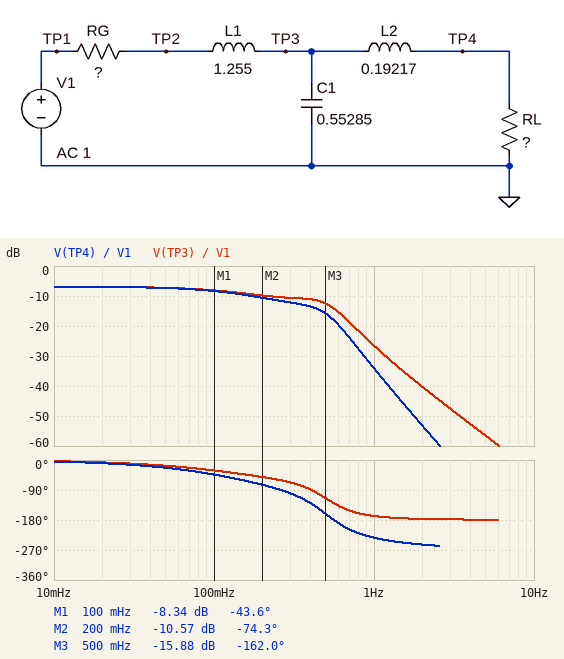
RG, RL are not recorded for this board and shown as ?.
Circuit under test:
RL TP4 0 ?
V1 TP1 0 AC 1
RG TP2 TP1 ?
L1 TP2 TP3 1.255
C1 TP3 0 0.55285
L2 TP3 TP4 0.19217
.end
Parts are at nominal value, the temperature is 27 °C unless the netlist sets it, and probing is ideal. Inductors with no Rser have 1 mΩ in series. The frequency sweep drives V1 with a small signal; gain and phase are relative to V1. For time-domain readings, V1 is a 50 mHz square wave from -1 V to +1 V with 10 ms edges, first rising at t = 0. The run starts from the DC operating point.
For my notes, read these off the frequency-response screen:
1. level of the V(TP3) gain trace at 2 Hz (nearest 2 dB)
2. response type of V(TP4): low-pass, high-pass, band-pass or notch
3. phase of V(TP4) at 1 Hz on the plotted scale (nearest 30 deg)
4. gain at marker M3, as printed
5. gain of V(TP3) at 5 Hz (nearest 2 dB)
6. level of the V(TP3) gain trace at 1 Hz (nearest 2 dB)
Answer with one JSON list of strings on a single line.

["-40 dB", "low-pass", "-240 deg", "-15.88 dB", "-56 dB", "-26 dB"]
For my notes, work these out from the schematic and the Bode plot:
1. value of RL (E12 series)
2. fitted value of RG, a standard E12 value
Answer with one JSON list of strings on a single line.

["0.56 Ω", "0.68 Ω"]
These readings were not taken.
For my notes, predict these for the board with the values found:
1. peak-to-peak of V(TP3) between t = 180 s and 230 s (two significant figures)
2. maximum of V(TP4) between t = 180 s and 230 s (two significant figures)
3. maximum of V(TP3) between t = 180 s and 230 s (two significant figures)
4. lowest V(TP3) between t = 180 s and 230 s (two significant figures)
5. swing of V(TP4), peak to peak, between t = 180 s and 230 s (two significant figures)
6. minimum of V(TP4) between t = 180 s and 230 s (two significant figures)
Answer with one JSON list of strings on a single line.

["900 mV", "450 mV", "450 mV", "-450 mV", "900 mV", "-450 mV"]
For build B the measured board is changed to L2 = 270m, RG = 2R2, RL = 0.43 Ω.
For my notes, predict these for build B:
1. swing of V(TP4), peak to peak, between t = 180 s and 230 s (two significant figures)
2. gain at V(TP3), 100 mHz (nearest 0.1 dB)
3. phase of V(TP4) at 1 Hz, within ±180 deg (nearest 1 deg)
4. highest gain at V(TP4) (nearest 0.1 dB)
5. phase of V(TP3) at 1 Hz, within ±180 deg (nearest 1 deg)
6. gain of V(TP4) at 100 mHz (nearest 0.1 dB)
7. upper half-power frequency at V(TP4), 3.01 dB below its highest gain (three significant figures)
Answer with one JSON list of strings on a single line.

["400 mV", "-15.3 dB", "123 deg", "-15.4 dB", "-161 deg", "-15.9 dB", "498 mHz"]
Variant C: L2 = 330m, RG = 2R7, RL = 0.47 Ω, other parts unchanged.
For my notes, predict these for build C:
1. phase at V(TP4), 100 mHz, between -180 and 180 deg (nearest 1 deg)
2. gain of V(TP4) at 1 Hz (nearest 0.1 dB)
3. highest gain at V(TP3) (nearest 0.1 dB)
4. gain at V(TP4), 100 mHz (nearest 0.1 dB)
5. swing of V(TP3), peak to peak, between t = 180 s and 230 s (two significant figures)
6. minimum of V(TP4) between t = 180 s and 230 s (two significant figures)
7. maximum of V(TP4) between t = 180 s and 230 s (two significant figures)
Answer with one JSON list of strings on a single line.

["-26 deg", "-40.8 dB", "-9.6 dB", "-16.6 dB", "630 mV", "-200 mV", "200 mV"]
